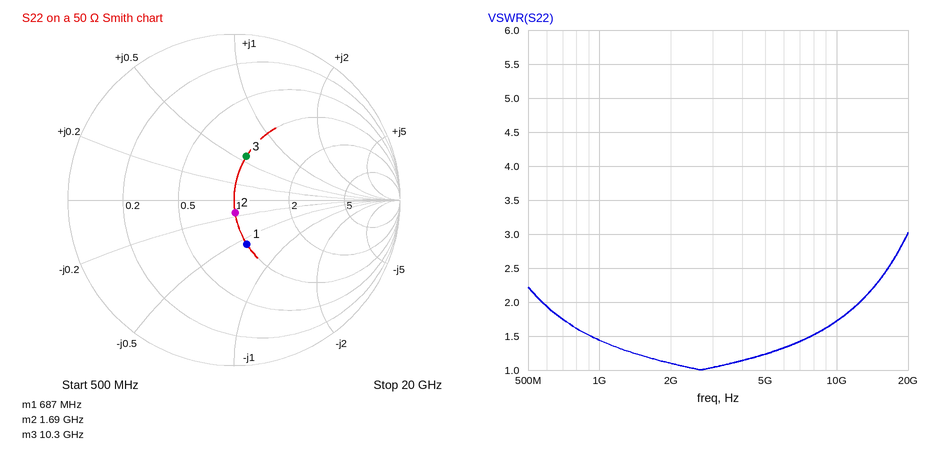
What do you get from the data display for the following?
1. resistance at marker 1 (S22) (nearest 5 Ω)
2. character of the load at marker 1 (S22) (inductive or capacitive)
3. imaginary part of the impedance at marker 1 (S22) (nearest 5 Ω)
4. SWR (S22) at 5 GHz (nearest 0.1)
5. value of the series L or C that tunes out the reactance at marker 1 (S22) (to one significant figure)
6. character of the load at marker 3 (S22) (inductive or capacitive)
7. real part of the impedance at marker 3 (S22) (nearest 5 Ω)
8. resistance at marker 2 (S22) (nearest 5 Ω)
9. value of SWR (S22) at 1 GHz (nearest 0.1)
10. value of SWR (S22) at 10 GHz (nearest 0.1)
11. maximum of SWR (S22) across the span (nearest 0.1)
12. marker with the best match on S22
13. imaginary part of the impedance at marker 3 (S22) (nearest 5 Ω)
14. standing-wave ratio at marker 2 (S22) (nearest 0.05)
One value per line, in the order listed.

50 Ω
capacitive
-30 Ω
1.2
7 nH
inductive
50 Ω
50 Ω
1.4
1.7
3.0
marker 2
+30 Ω
1.15
